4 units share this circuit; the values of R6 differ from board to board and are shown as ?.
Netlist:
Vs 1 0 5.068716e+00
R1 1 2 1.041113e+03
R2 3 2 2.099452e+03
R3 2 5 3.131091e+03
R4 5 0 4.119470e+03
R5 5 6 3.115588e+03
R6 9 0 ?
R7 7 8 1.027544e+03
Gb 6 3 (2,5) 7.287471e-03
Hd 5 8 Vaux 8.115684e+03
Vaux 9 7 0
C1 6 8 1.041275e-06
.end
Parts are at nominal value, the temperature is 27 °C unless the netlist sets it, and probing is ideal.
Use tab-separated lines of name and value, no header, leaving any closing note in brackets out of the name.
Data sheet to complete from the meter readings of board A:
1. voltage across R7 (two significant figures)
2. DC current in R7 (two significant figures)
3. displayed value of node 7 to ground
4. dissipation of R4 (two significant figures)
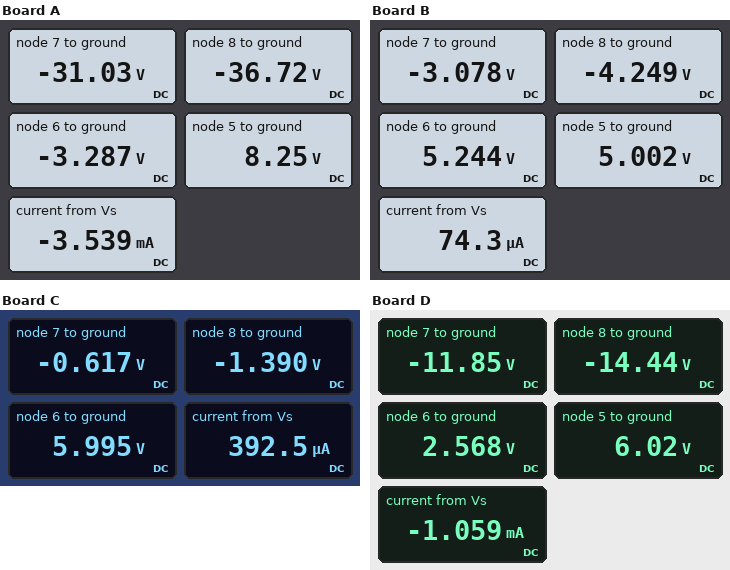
voltage across R7	5.7 V
DC current in R7	5.5 mA
displayed value of node 7 to ground	-31.03 V
dissipation of R4	17 mW
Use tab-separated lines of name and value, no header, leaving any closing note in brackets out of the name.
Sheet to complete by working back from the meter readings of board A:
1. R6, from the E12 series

R6, from the E12 series	5.6 kΩ
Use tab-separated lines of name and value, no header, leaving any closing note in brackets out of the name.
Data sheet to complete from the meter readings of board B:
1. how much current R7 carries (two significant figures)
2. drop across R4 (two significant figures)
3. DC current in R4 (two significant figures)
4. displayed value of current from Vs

how much current R7 carries	1.1 mA
drop across R4	5.0 V
DC current in R4	1.2 mA
displayed value of current from Vs	74.3 µA
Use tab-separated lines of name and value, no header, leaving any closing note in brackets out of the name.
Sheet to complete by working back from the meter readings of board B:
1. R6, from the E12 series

R6, from the E12 series	2.7 kΩ
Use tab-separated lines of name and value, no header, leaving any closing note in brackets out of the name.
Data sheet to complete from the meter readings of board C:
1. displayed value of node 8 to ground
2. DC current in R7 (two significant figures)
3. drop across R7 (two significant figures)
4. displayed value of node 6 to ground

displayed value of node 8 to ground	-1.390 V
DC current in R7	750 µA
drop across R7	770 mV
displayed value of node 6 to ground	5.995 V
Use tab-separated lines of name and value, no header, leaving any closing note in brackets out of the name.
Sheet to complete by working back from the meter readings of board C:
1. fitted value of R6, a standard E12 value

fitted value of R6, a standard E12 value	820 Ω
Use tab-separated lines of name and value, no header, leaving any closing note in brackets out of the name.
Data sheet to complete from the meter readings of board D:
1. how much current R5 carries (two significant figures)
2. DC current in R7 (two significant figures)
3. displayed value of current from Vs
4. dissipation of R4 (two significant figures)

how much current R5 carries	1.1 mA
DC current in R7	2.5 mA
displayed value of current from Vs	-1.059 mA
dissipation of R4	8.8 mW
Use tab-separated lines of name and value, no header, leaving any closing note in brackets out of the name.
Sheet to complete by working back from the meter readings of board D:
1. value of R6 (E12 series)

value of R6	4.7 kΩ
